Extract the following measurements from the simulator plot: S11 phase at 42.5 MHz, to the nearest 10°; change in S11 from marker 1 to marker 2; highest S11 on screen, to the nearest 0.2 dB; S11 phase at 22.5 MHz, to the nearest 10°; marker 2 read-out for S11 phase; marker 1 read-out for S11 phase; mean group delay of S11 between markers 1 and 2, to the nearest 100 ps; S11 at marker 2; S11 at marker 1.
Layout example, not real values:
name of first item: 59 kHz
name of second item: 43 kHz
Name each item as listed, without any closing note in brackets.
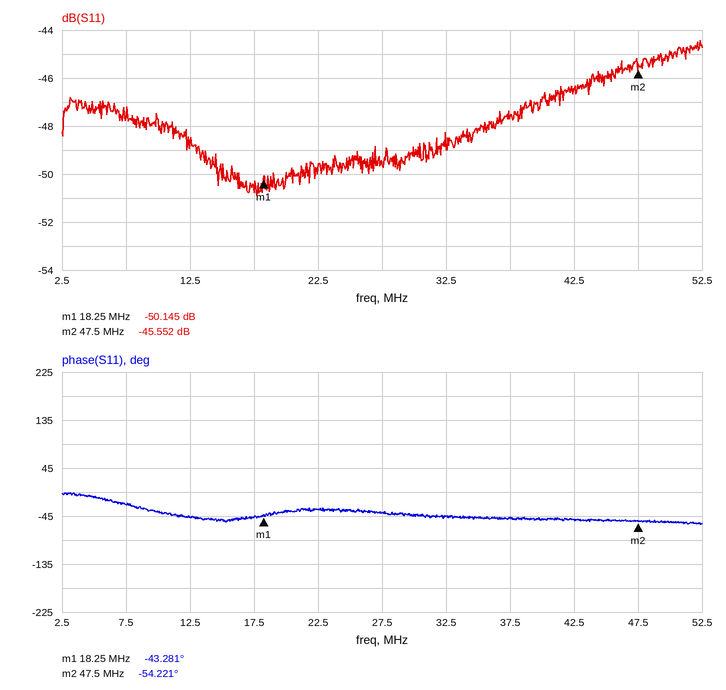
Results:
S11 phase at 42.5 MHz, to the nearest 10°: -50°
change in S11 from marker 1 to marker 2: 4.593 dB
highest S11 on screen, to the nearest 0.2 dB: -44.4 dB
S11 phase at 22.5 MHz, to the nearest 10°: -30°
marker 2 read-out for S11 phase: -54.221°
marker 1 read-out for S11 phase: -43.281°
mean group delay of S11 between markers 1 and 2, to the nearest 100 ps: 1.0 ns
S11 at marker 2: -45.552 dB
S11 at marker 1: -50.145 dB
